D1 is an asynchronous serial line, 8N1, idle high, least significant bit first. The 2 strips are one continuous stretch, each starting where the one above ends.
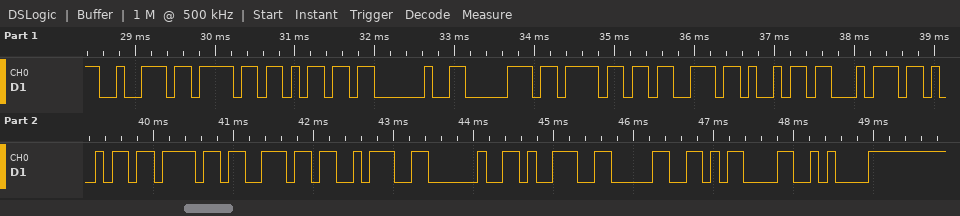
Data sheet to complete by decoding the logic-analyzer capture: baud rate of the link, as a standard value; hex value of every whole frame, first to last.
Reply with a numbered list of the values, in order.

1. 9600 baud
2. 0x72 0x6F 0x6D 0x20 0x70 0x6F 0x73 0x69 0x74 0x69 0x6F 0x6E 0x3A 0x20 0x39 0x30 0x0D 0x0A
